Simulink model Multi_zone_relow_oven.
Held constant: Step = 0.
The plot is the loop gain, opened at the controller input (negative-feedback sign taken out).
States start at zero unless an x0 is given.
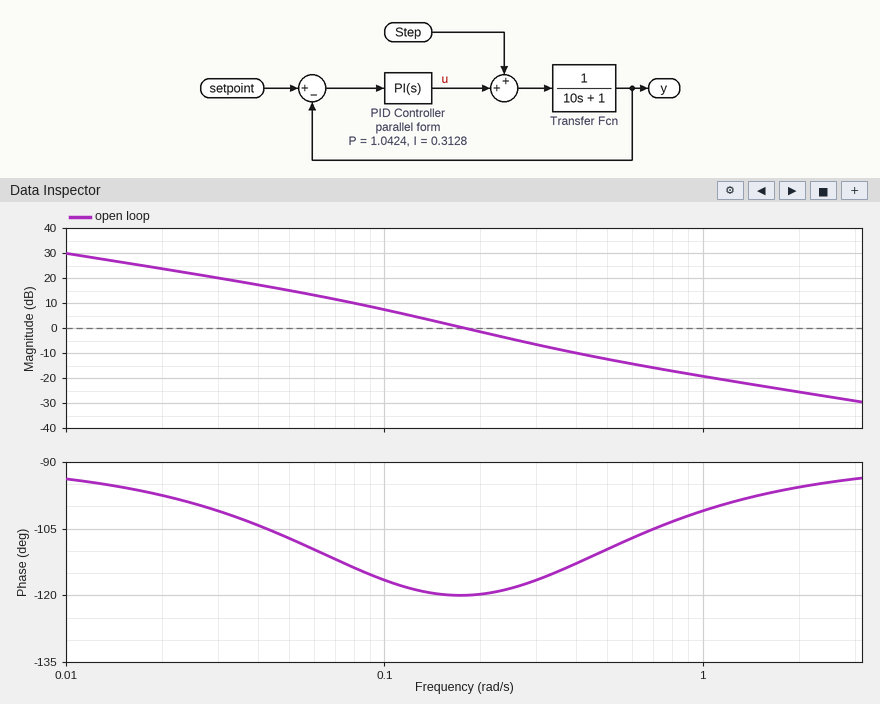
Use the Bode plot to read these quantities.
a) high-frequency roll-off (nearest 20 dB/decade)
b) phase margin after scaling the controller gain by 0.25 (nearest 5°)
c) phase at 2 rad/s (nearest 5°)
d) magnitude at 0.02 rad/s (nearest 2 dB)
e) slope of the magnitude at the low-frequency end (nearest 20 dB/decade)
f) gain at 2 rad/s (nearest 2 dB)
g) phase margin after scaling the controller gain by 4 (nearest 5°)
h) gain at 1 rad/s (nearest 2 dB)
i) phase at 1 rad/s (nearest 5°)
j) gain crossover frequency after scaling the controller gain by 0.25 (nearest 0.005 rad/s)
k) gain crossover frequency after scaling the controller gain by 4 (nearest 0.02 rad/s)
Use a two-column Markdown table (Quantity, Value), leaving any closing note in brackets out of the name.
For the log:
| Quantity | Value |
|---|---|
| high-frequency roll-off | -20 dB/decade |
| phase margin after scaling the controller gain by 0.25 | 70° |
| phase at 2 rad/s | -95° |
| magnitude at 0.02 rad/s | 24 dB |
| slope of the magnitude at the low-frequency end | -20 dB/decade |
| gain at 2 rad/s | -26 dB |
| phase margin after scaling the controller gain by 4 | 70° |
| gain at 1 rad/s | -20 dB |
| phase at 1 rad/s | -100° |
| gain crossover frequency after scaling the controller gain by 0.25 | 0.065 rad/s |
| gain crossover frequency after scaling the controller gain by 4 | 0.48 rad/s |
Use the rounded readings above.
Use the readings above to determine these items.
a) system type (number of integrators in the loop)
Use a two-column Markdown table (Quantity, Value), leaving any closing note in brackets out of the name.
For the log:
| Quantity | Value |
|---|---|
| system type | 1 |
